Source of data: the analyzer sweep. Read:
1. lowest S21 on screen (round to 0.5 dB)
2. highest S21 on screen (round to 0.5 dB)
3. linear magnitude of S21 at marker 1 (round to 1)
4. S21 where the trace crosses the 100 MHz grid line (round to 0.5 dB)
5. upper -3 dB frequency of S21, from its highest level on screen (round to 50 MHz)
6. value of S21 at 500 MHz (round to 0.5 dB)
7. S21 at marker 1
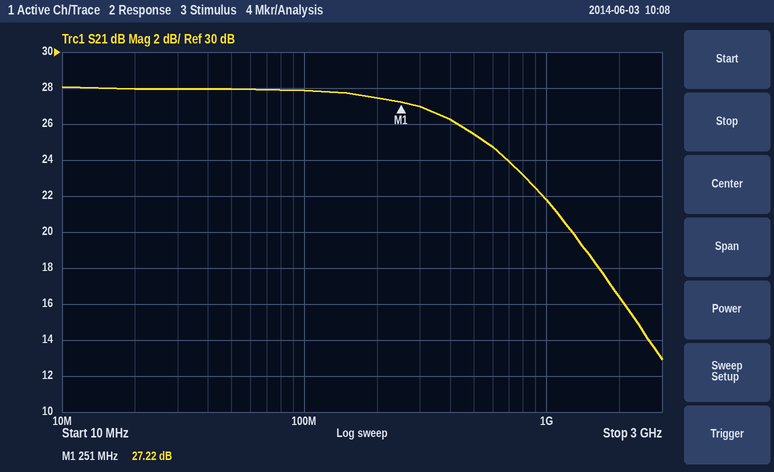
13.0 dB
28.0 dB
23
28.0 dB
550 MHz
25.5 dB
27.22 dB
